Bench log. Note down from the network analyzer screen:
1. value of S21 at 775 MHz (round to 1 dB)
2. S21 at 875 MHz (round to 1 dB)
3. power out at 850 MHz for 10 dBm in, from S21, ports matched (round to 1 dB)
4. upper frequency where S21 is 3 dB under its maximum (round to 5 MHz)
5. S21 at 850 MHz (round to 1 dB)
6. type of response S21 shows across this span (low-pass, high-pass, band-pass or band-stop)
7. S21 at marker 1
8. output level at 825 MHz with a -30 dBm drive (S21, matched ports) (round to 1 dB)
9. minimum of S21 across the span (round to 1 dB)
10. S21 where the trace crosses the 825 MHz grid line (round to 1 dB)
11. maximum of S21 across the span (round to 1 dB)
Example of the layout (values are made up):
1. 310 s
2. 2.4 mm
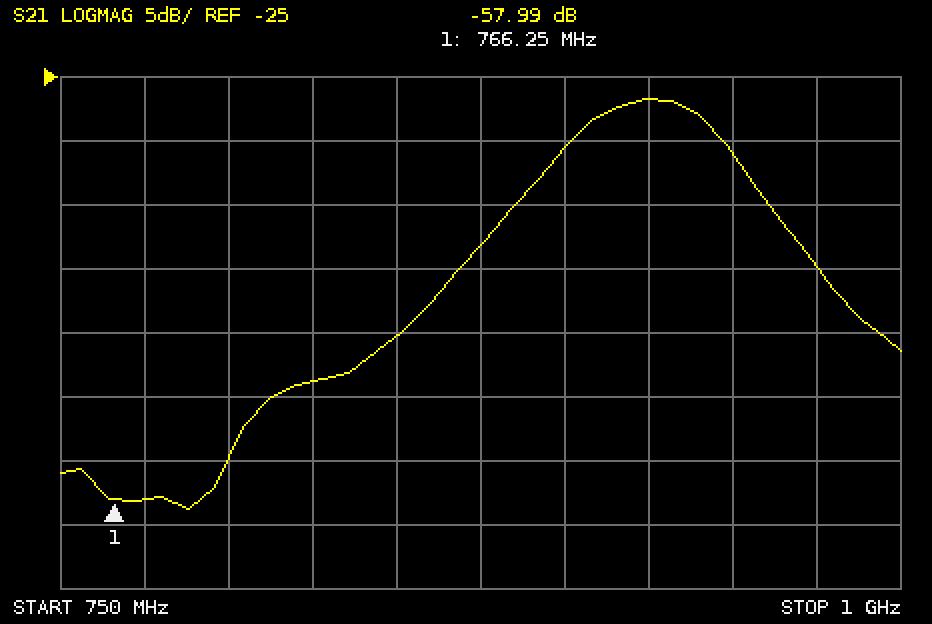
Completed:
1. -58 dB
2. -38 dB
3. -35 dBm
4. 945 MHz
5. -45 dB
6. band-pass
7. -57.99 dB
8. -79 dBm
9. -59 dB
10. -49 dB
11. -27 dB
